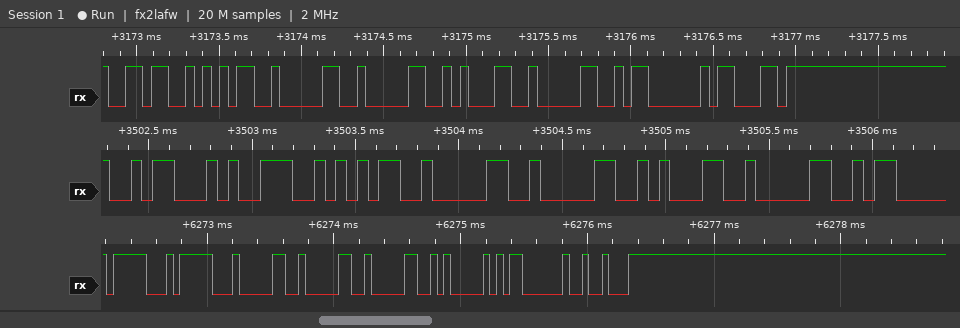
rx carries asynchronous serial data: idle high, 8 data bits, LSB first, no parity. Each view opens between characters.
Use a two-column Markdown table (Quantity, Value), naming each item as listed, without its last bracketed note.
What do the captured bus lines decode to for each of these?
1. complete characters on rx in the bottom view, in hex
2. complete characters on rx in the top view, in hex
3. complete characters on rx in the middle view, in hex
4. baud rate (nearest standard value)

| Quantity | Value |
|---|---|
| complete characters on rx in the bottom view, in hex | 1F, 1F, 30, 30, 30, 41, 03, 12 |
| complete characters on rx in the top view, in hex | 36, 35, 30, 30, 31, 30, 03, 63 |
| complete characters on rx in the middle view, in hex | 1A, 39, 35, 30, 30, 31, 30 |
| baud rate | 19200 baud |
